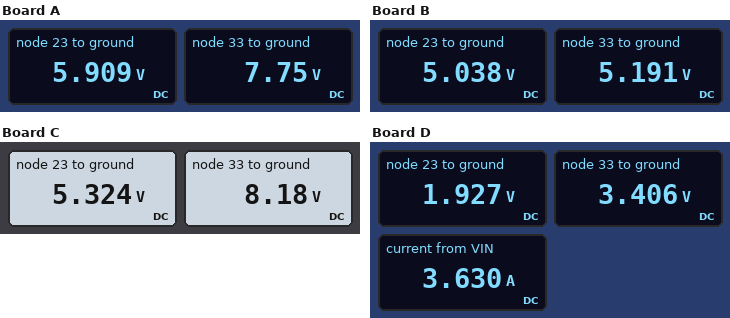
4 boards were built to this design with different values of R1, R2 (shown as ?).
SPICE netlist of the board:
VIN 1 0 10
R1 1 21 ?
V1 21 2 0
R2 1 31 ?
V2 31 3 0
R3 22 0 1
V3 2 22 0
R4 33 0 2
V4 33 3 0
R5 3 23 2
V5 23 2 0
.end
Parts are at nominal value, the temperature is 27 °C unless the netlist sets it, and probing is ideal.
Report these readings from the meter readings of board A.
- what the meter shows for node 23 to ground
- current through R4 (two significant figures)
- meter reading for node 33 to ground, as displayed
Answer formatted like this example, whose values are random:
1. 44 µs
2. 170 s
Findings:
1. 5.909 V
2. 3.9 A
3. 7.75 V
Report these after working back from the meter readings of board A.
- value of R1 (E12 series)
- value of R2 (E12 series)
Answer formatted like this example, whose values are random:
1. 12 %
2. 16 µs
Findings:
1. 0.82 Ω
2. 0.47 Ω
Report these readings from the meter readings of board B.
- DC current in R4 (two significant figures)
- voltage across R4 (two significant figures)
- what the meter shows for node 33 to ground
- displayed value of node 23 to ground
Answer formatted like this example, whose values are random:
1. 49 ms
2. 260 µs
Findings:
1. 2.6 A
2. 5.2 V
3. 5.191 V
4. 5.038 V
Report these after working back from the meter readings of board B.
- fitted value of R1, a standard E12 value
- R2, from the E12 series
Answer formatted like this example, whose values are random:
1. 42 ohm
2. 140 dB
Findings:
1. 1 Ω
2. 1.8 Ω
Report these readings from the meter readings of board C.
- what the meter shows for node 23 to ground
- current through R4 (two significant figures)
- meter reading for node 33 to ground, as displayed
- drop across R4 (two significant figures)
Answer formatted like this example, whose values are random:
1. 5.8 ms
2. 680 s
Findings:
1. 5.324 V
2. 4.1 A
3. 8.18 V
4. 8.2 V
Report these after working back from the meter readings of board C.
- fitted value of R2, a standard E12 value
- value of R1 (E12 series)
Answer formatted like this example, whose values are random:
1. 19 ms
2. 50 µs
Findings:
1. 0.33 Ω
2. 1.2 Ω
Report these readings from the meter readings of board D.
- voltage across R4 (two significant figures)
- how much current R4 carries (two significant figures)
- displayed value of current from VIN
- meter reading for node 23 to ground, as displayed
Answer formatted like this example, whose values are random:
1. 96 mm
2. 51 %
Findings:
1. 3.4 V
2. 1.7 A
3. 3.630 A
4. 1.927 V
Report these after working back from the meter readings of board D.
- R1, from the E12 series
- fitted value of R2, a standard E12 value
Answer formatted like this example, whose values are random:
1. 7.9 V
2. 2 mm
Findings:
1. 6.8 Ω
2. 2.7 Ω
